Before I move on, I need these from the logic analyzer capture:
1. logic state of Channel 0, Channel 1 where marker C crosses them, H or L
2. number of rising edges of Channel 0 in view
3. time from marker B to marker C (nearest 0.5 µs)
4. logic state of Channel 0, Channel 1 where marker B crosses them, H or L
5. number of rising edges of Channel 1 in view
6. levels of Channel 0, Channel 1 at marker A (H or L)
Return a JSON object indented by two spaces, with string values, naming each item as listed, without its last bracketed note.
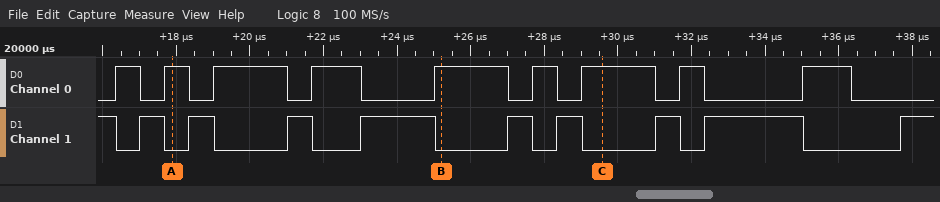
{
  "logic state of Channel 0, Channel 1 where marker C crosses them, H or L": "Channel 0=H, Channel 1=L",
  "number of rising edges of Channel 0 in view": "9",
  "time from marker B to marker C": "4.5 µs",
  "logic state of Channel 0, Channel 1 where marker B crosses them, H or L": "Channel 0=H, Channel 1=L",
  "number of rising edges of Channel 1 in view": "9",
  "levels of Channel 0, Channel 1 at marker A": "Channel 0=H, Channel 1=L"
}
